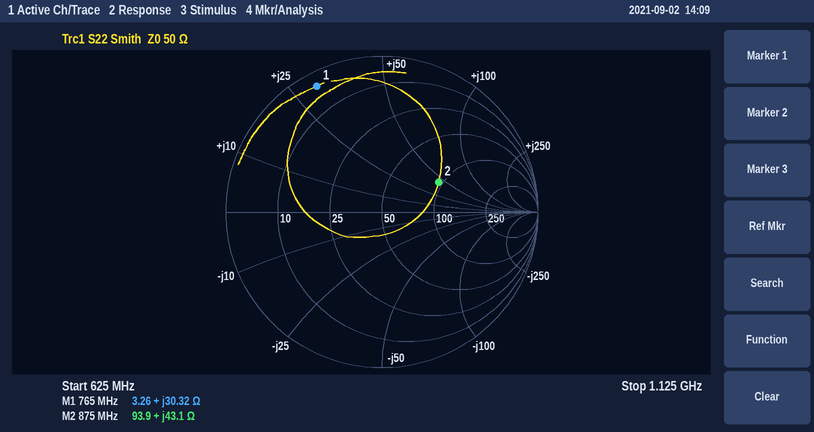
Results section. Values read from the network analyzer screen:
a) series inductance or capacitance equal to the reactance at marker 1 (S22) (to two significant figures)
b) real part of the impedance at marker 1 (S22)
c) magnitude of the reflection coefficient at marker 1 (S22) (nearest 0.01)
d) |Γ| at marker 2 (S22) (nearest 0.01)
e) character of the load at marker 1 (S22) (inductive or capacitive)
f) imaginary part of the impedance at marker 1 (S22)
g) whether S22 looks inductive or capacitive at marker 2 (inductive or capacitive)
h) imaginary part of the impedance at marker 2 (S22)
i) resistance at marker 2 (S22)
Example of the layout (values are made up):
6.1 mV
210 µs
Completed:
6.3 nH
3.26 Ω
0.91
0.41
inductive
+30.32 Ω
inductive
+43.1 Ω
93.9 Ω
